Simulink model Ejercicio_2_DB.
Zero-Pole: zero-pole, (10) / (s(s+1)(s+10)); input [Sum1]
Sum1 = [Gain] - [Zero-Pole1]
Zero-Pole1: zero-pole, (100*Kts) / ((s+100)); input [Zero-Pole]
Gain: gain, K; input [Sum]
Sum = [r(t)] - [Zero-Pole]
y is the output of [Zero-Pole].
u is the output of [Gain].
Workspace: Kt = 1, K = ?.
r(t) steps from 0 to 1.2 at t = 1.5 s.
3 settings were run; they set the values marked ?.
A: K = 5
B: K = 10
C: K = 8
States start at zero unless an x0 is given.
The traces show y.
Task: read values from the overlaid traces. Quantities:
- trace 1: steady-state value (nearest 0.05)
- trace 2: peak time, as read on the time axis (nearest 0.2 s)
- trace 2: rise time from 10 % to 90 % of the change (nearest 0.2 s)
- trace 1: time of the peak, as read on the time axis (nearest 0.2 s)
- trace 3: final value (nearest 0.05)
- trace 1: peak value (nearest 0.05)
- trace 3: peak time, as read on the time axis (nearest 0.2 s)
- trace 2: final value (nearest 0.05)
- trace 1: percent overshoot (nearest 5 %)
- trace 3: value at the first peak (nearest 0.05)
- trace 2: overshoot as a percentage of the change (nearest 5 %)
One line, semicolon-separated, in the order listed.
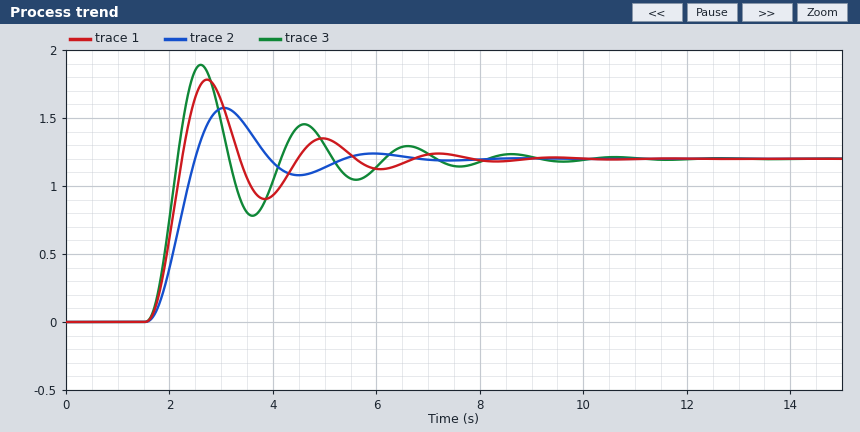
1.20; 3.0 s; 0.6 s; 2.8 s; 1.20; 1.80; 2.6 s; 1.20; 50 %; 1.90; 30 %
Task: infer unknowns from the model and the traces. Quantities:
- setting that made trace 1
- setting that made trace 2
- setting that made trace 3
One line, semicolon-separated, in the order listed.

C; A; B
